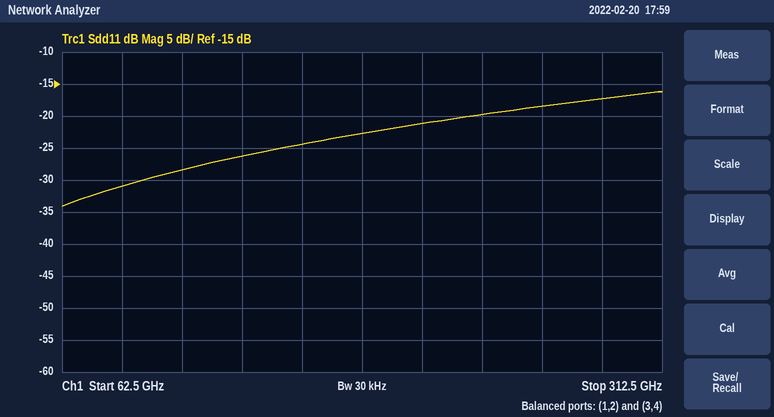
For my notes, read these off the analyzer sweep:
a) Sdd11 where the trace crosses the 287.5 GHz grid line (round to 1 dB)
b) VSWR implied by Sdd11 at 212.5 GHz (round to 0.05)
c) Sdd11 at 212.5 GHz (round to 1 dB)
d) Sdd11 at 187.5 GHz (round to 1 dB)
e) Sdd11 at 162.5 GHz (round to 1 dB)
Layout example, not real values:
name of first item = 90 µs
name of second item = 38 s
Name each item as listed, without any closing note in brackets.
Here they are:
Sdd11 where the trace crosses the 287.5 GHz grid line = -17 dB
VSWR implied by Sdd11 at 212.5 GHz = 1.20
Sdd11 at 212.5 GHz = -21 dB
Sdd11 at 187.5 GHz = -23 dB
Sdd11 at 162.5 GHz = -24 dB
